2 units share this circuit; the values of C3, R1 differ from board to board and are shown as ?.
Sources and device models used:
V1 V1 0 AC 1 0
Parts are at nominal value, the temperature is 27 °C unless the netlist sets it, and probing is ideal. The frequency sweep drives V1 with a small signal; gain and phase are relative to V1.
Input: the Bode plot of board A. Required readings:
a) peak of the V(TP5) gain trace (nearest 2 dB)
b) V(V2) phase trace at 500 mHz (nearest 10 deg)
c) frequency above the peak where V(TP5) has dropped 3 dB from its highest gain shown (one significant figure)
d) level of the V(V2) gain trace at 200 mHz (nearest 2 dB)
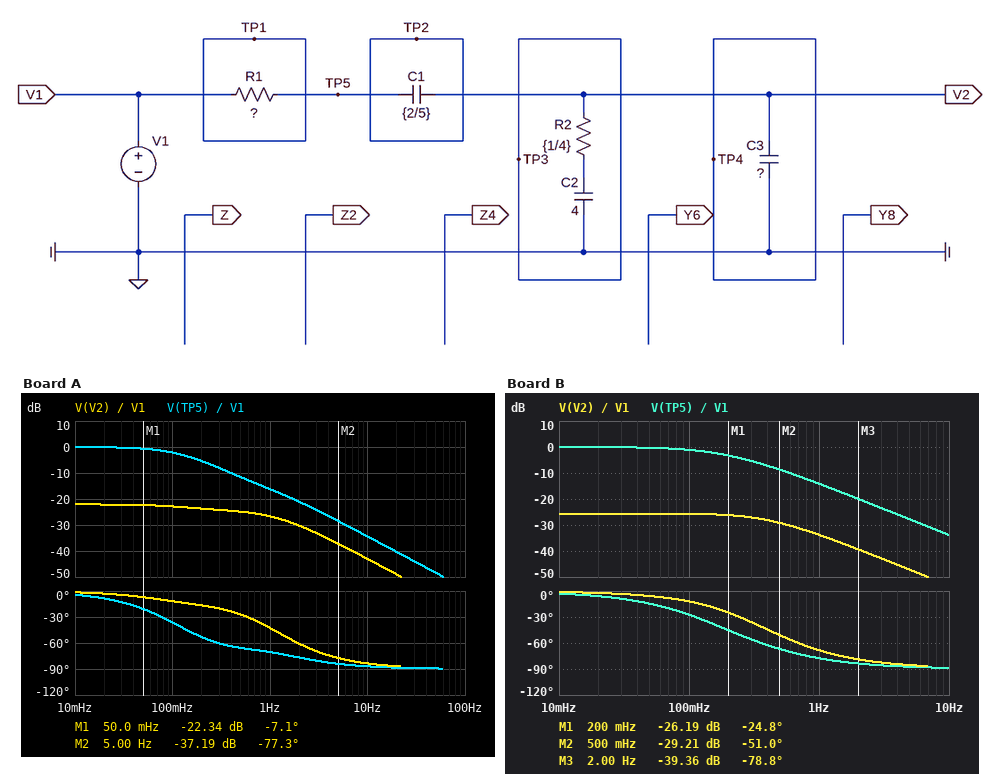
0 dB
-30 deg
100 mHz
-24 dB
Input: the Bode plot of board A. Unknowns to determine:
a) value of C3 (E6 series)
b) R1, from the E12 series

680 mF
3.3 Ω
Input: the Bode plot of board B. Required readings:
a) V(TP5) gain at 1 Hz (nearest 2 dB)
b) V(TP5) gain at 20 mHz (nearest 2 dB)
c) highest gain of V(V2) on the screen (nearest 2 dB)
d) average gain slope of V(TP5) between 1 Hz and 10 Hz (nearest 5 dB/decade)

-14 dB
0 dB
-26 dB
-20 dB/decade
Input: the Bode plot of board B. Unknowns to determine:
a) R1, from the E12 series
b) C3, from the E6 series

2.2 Ω
3.3 F
